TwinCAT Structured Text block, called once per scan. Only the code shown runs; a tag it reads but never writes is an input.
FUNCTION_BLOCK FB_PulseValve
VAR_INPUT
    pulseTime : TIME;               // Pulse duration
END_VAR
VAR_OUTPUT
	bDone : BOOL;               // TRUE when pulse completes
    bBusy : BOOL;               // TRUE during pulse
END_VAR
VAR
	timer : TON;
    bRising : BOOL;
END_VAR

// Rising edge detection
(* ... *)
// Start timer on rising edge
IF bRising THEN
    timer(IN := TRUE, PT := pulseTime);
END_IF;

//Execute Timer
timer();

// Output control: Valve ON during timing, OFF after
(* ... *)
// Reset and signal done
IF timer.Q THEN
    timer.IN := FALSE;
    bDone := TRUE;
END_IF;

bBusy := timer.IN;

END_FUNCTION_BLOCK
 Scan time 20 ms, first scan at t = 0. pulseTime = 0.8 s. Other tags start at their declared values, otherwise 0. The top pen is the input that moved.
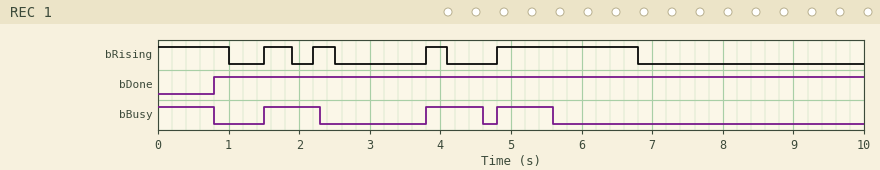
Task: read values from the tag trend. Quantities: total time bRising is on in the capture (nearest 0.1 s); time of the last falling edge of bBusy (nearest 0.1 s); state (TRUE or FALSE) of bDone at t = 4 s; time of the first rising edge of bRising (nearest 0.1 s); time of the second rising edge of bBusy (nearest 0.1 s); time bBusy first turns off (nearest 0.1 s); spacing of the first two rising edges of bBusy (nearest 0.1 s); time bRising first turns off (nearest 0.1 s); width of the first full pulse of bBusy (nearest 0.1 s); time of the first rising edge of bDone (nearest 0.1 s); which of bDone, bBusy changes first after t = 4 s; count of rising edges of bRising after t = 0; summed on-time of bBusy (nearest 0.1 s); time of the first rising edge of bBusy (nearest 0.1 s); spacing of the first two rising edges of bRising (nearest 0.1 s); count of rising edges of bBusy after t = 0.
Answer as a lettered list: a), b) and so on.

a) 4.0 s
b) 5.6 s
c) TRUE
d) 1.5 s
e) 3.8 s
f) 0.8 s
g) 2.3 s
h) 1.0 s
i) 0.8 s
j) 0.8 s
k) bBusy
l) 4
m) 3.2 s
n) 1.5 s
o) 0.7 s
p) 3
